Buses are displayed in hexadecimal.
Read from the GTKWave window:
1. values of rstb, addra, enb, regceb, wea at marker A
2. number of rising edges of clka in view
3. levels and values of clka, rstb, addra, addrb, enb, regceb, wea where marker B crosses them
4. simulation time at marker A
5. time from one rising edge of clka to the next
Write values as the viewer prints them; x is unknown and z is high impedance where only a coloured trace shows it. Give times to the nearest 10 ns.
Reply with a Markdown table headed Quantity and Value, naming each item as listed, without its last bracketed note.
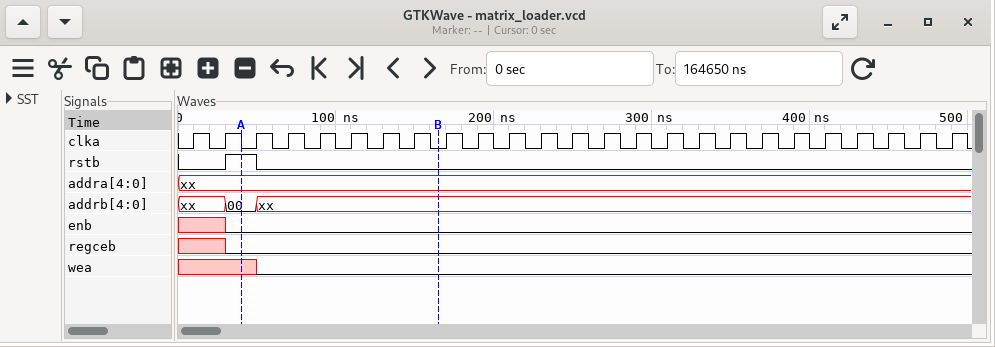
| Quantity | Value |
|---|---|
| values of rstb, addra, enb, regceb, wea at marker A | rstb=1, addra=xx, enb=0, regceb=0, wea=x |
| number of rising edges of clka in view | 25 |
| levels and values of clka, rstb, addra, addrb, enb, regceb, wea where marker B crosses them | clka=0, rstb=0, addra=xx, addrb=xx, enb=0, regceb=0, wea=0 |
| simulation time at marker A | 40 ns |
| time from one rising edge of clka to the next | 20 ns |
